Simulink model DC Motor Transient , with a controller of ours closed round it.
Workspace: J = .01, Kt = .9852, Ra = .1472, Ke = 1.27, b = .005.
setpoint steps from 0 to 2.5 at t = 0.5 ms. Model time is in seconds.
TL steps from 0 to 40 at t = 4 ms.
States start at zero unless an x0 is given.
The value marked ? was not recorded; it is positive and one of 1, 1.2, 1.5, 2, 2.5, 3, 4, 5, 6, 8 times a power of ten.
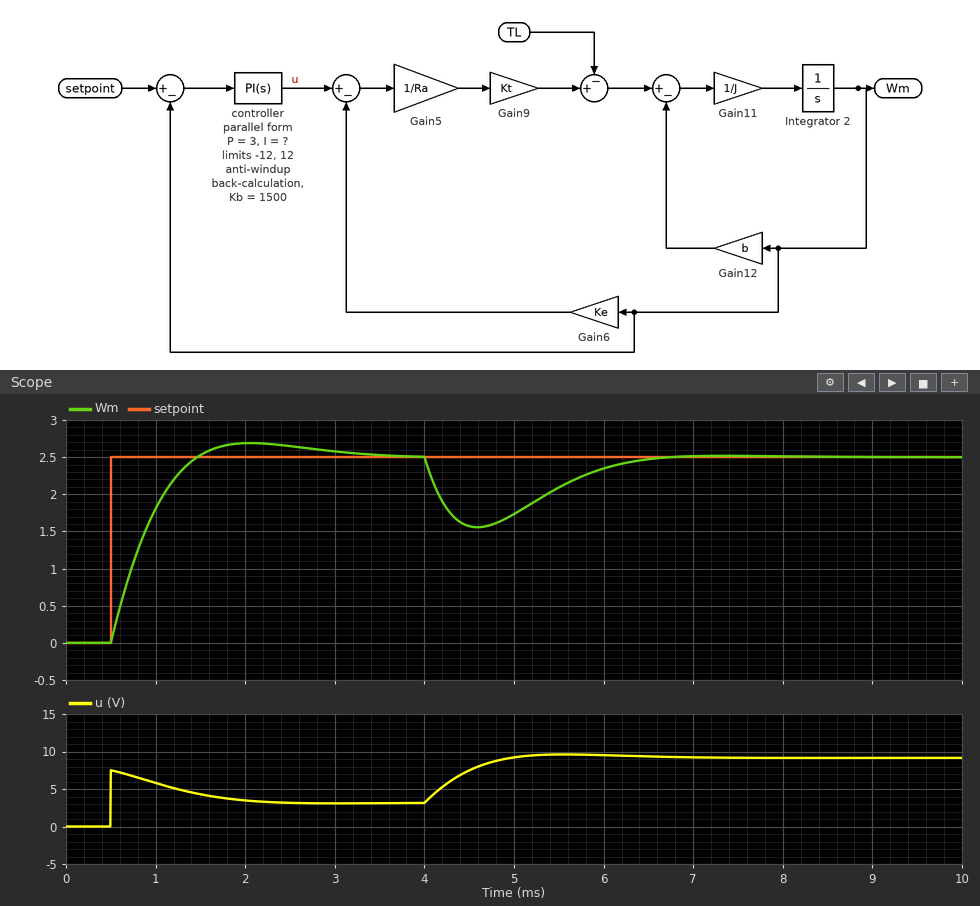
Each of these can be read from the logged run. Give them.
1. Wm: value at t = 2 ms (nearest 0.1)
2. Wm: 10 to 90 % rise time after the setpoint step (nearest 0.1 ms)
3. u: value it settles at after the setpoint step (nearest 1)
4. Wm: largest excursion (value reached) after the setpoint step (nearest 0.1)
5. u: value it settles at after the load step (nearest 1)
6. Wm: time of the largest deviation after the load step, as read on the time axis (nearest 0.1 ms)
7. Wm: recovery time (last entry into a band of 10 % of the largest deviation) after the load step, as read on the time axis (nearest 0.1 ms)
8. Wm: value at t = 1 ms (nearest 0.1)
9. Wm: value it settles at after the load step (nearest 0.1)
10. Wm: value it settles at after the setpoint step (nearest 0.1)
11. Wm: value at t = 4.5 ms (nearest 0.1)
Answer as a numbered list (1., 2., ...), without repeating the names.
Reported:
1. 2.7
2. 0.7 ms
3. 3
4. 2.7
5. 9
6. 4.6 ms
7. 6.2 ms
8. 1.8
9. 2.5
10. 2.5
11. 1.6
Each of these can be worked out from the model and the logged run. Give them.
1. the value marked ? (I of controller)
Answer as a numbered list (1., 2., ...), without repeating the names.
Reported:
1. 5000
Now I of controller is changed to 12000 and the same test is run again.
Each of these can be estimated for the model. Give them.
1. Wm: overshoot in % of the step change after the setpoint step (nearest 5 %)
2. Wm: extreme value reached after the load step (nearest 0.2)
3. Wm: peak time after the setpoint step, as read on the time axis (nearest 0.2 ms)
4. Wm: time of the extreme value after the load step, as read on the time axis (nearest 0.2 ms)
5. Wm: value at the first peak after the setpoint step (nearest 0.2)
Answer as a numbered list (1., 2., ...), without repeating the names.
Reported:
1. 20 %
2. 1.8
3. 1.4 ms
4. 4.4 ms
5. 3.0
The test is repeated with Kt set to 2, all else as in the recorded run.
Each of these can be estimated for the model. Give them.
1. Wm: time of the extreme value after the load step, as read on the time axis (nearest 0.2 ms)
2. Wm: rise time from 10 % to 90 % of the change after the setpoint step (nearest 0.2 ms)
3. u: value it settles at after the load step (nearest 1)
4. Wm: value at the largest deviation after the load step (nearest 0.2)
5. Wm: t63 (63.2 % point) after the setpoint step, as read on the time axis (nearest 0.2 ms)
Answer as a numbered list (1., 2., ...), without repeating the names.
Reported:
1. 4.4 ms
2. 0.6 ms
3. 6
4. 2.0
5. 0.8 ms
